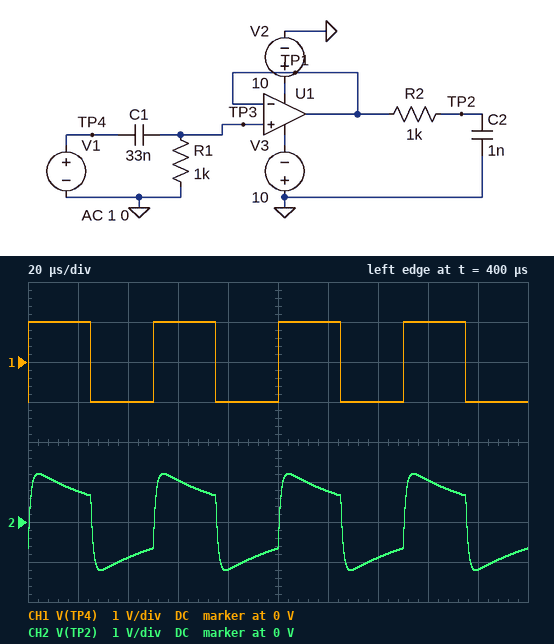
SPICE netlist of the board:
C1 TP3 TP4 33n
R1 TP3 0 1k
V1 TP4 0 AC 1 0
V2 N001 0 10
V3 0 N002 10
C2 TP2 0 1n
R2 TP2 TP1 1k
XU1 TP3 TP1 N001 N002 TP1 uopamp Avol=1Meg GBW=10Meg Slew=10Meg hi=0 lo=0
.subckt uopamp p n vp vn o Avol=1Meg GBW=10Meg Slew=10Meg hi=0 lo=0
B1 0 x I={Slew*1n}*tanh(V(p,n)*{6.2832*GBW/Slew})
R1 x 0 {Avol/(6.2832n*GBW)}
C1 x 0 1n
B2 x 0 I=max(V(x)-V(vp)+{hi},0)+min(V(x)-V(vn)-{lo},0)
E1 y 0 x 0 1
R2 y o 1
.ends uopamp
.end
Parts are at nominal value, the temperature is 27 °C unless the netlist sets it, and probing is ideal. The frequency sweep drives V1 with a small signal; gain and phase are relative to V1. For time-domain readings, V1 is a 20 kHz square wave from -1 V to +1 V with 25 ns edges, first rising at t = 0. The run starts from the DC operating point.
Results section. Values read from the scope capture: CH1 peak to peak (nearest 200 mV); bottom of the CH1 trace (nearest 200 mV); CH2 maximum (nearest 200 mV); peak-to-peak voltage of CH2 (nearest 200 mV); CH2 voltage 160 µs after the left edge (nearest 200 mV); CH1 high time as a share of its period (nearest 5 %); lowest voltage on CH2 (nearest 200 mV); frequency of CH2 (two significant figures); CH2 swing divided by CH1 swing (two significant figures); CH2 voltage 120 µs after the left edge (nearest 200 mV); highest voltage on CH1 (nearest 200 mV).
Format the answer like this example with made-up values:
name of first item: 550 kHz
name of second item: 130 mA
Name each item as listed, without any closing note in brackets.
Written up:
CH1 peak to peak: 2.0 V
bottom of the CH1 trace: -1.0 V
CH2 maximum: 1.2 V
peak-to-peak voltage of CH2: 2.4 V
CH2 voltage 160 µs after the left edge: 1.0 V
CH1 high time as a share of its period: 50 %
lowest voltage on CH2: -1.2 V
frequency of CH2: 20 kHz
CH2 swing divided by CH1 swing: 1.2
CH2 voltage 120 µs after the left edge: 800 mV
highest voltage on CH1: 1.0 V
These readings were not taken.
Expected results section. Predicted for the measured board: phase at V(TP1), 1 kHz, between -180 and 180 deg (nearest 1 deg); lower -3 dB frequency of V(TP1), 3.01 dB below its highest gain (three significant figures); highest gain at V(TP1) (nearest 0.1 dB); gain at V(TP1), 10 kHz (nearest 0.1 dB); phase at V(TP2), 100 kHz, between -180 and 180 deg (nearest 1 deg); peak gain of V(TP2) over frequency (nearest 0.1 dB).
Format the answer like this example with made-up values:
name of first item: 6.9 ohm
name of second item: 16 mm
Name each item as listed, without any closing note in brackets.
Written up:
phase at V(TP1), 1 kHz, between -180 and 180 deg: 78 deg
lower -3 dB frequency of V(TP1), 3.01 dB below its highest gain: 4.82 kHz
highest gain at V(TP1): 0 dB
gain at V(TP1), 10 kHz: -0.9 dB
phase at V(TP2), 100 kHz, between -180 and 180 deg: -30 deg
peak gain of V(TP2) over frequency: -0.3 dB
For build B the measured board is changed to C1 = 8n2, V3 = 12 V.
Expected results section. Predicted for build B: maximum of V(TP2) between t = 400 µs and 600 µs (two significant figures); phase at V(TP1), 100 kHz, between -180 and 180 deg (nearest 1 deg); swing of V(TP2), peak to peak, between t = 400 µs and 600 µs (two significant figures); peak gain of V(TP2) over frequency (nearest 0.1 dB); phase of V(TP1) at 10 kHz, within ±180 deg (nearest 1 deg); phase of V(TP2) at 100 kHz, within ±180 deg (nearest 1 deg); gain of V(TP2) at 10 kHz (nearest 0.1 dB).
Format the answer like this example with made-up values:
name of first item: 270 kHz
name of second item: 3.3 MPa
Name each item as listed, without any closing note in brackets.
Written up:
maximum of V(TP2) between t = 400 µs and 600 µs: 1.4 V
phase at V(TP1), 100 kHz, between -180 and 180 deg: 10 deg
swing of V(TP2), peak to peak, between t = 400 µs and 600 µs: 2.8 V
peak gain of V(TP2) over frequency: -1.0 dB
phase of V(TP1) at 10 kHz, within ±180 deg: 63 deg
phase of V(TP2) at 100 kHz, within ±180 deg: -22 deg
gain of V(TP2) at 10 kHz: -6.8 dB
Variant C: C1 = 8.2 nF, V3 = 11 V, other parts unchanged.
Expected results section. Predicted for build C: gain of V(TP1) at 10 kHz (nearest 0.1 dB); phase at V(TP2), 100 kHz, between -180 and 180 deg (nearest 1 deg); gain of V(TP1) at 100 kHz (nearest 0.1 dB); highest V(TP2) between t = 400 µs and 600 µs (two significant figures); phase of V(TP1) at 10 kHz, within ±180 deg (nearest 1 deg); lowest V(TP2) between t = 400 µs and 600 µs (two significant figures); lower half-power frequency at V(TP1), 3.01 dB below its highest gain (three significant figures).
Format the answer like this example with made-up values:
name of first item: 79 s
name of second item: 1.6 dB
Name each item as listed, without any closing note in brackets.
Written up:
gain of V(TP1) at 10 kHz: -6.8 dB
phase at V(TP2), 100 kHz, between -180 and 180 deg: -22 deg
gain of V(TP1) at 100 kHz: -0.2 dB
highest V(TP2) between t = 400 µs and 600 µs: 1.4 V
phase of V(TP1) at 10 kHz, within ±180 deg: 63 deg
lowest V(TP2) between t = 400 µs and 600 µs: -1.4 V
lower half-power frequency at V(TP1), 3.01 dB below its highest gain: 19.3 kHz
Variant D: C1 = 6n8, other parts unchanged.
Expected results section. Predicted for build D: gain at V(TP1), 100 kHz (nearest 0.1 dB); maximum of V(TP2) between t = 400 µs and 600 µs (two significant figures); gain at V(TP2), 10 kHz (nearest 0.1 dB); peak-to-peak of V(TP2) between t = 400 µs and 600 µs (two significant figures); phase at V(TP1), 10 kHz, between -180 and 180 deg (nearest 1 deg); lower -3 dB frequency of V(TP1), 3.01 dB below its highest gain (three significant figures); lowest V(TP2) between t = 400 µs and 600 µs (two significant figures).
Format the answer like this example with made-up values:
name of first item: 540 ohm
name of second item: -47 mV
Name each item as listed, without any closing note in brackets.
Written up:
gain at V(TP1), 100 kHz: -0.2 dB
maximum of V(TP2) between t = 400 µs and 600 µs: 1.4 V
gain at V(TP2), 10 kHz: -8.1 dB
peak-to-peak of V(TP2) between t = 400 µs and 600 µs: 2.8 V
phase at V(TP1), 10 kHz, between -180 and 180 deg: 67 deg
lower -3 dB frequency of V(TP1), 3.01 dB below its highest gain: 23.3 kHz
lowest V(TP2) between t = 400 µs and 600 µs: -1.4 V
